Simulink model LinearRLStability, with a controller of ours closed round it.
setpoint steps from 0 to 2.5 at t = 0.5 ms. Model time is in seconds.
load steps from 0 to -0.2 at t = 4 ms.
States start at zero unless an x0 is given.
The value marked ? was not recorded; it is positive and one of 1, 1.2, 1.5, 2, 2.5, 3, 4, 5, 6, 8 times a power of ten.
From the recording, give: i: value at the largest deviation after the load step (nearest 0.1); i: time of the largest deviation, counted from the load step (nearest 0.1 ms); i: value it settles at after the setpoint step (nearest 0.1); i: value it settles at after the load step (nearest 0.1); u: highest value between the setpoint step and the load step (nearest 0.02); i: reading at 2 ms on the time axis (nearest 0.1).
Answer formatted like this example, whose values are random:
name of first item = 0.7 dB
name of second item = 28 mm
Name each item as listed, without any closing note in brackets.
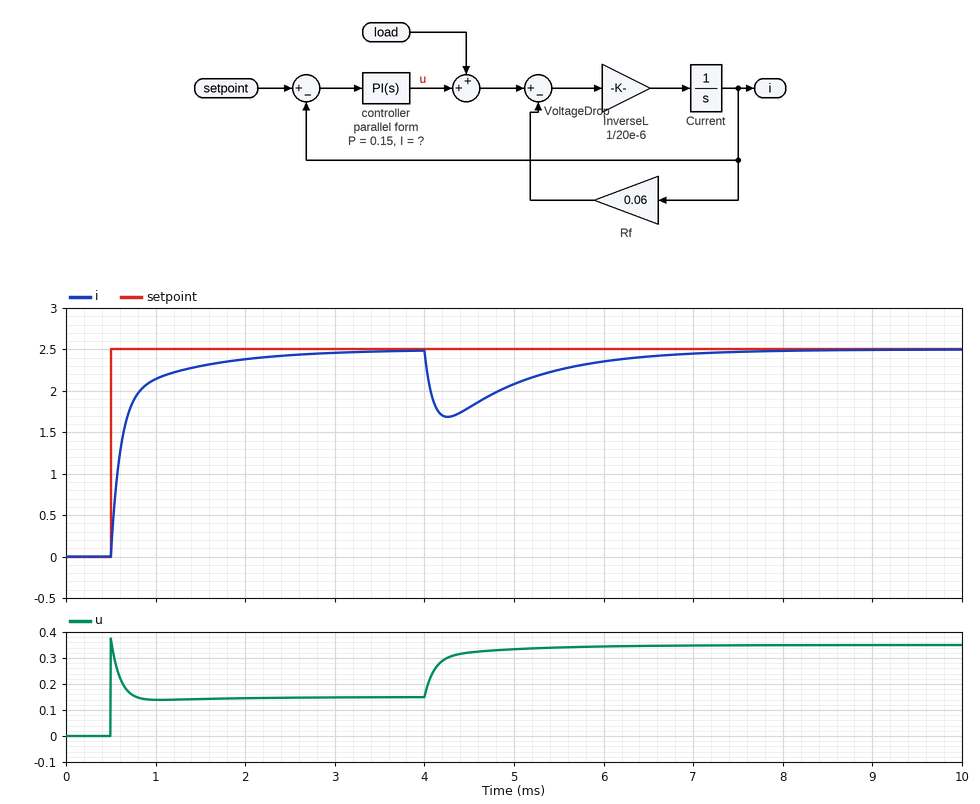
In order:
i: value at the largest deviation after the load step = 1.7
i: time of the largest deviation, counted from the load step = 0.3 ms
i: value it settles at after the setpoint step = 2.5
i: value it settles at after the load step = 2.5
u: highest value between the setpoint step and the load step = 0.38
i: reading at 2 ms on the time axis = 2.4
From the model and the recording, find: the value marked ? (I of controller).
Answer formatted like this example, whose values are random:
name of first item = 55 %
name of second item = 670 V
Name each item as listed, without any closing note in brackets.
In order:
the value marked ? = 200
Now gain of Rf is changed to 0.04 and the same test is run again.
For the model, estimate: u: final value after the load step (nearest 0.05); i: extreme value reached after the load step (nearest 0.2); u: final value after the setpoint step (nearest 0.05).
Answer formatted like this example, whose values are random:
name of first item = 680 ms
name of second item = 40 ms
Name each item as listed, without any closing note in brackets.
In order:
u: final value after the load step = 0.30
i: extreme value reached after the load step = 1.6
u: final value after the setpoint step = 0.10
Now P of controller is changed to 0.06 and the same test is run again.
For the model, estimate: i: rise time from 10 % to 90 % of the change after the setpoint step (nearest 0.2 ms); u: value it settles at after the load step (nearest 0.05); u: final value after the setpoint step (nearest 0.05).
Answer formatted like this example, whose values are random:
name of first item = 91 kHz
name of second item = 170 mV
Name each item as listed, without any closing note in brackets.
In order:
i: rise time from 10 % to 90 % of the change after the setpoint step = 0.6 ms
u: value it settles at after the load step = 0.35
u: final value after the setpoint step = 0.15
